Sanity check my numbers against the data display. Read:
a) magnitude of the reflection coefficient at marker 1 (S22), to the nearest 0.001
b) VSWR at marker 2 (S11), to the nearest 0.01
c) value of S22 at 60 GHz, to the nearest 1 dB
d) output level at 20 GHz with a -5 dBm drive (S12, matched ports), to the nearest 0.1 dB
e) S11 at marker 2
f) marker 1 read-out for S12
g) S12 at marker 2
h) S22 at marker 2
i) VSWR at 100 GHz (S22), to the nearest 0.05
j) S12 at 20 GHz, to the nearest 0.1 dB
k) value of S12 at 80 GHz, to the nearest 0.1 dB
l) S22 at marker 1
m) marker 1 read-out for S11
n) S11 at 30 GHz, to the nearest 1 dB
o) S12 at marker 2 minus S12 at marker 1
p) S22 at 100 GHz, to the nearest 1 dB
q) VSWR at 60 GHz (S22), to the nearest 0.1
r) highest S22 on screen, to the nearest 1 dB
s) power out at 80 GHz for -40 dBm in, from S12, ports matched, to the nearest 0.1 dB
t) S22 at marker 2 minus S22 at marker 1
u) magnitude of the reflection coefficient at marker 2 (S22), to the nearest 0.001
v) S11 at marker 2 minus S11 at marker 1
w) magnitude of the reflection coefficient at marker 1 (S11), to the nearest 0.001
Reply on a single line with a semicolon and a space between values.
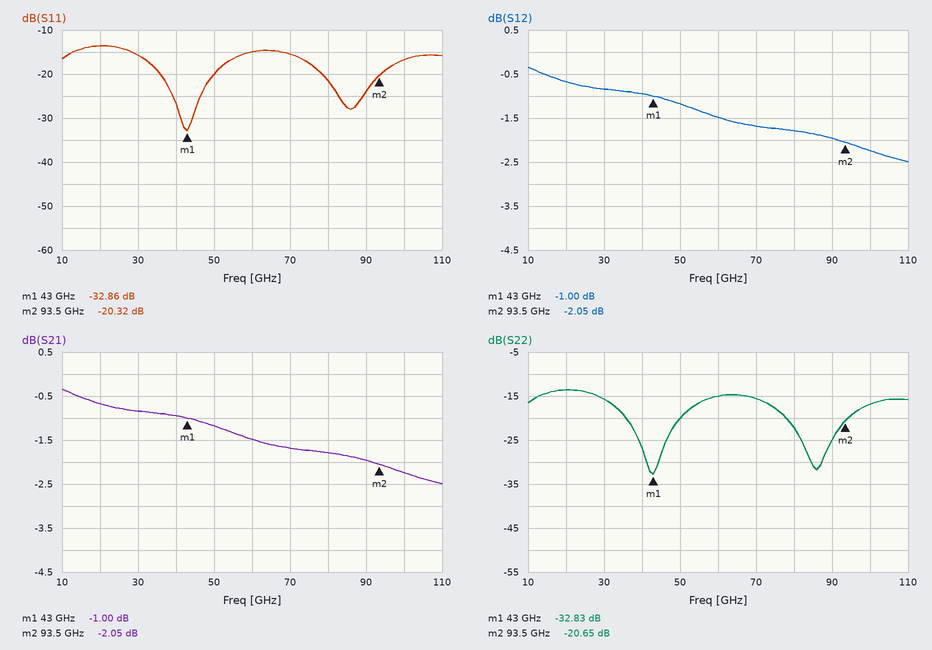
0.023; 1.21; -15 dB; -5.7 dBm; -20.32 dB; -1.00 dB; -2.05 dB; -20.65 dB; 1.35; -0.7 dB; -1.8 dB; -32.83 dB; -32.86 dB; -16 dB; -1.05 dB; -17 dB; 1.4; -14 dB; -41.8 dBm; 12.18 dB; 0.093; 12.54 dB; 0.023
